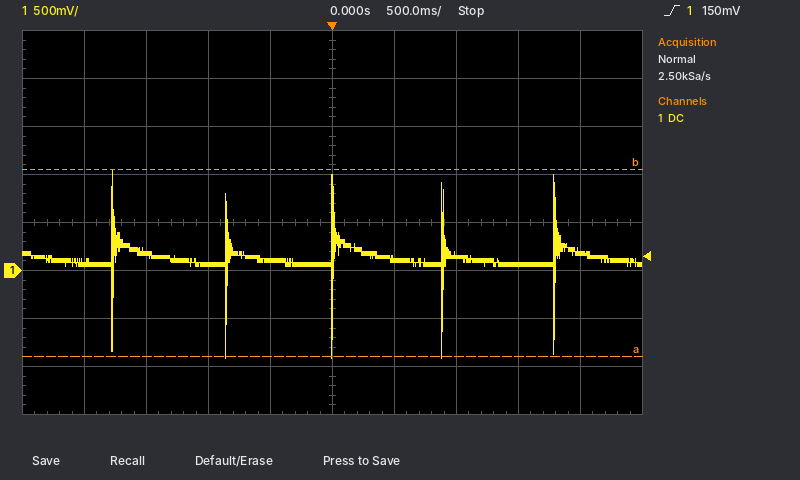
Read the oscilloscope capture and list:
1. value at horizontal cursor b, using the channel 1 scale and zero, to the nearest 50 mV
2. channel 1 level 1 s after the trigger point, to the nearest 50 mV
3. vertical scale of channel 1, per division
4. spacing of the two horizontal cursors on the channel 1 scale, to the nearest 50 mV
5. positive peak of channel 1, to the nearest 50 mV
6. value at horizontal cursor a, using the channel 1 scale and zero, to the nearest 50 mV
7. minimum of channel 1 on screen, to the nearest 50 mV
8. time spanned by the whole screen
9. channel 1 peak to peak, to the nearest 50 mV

1.05 V
150 mV
500 mV
1.95 V
1.05 V
-900 mV
-900 mV
5 s
1.95 V
